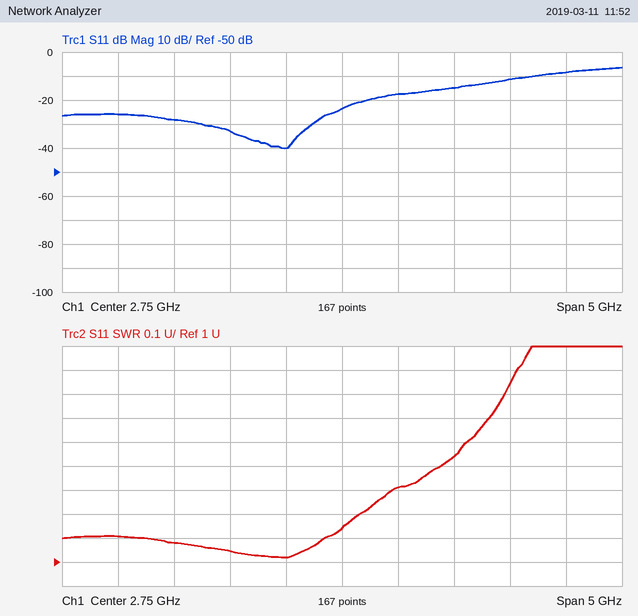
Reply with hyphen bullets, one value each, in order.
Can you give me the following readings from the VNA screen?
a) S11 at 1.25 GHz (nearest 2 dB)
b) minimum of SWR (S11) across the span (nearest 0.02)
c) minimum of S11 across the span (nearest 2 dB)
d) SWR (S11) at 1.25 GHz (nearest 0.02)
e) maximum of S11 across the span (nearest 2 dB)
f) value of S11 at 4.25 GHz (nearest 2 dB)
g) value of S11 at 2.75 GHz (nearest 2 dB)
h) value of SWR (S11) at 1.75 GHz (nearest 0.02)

- -28 dB
- 1.02
- -40 dB
- 1.08
- -6 dB
- -12 dB
- -24 dB
- 1.04
